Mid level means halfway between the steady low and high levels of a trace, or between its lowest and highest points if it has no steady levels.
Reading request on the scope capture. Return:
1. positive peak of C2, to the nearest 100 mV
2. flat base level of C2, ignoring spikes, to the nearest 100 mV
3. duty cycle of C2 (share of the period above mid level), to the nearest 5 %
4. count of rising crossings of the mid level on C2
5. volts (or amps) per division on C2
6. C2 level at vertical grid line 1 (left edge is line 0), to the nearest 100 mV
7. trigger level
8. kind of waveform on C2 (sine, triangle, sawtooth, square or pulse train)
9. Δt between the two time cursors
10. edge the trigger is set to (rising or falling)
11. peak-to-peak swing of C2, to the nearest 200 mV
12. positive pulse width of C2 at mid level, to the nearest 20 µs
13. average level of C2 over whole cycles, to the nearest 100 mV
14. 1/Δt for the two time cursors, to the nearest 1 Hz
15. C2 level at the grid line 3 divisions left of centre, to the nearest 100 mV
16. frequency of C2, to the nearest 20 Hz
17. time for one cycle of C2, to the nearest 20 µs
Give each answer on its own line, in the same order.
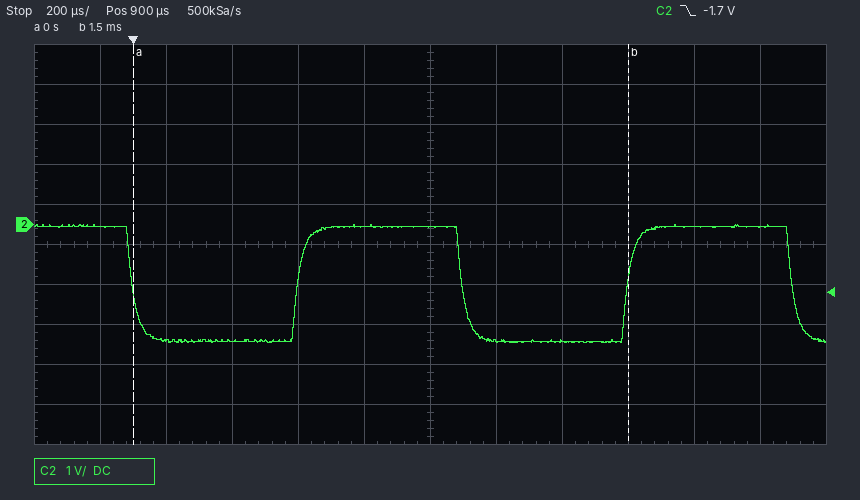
0.0 V
-2.9 V
50 %
2
1 V
0.0 V
-1.7 V
square
1.50 ms
falling
3.0 V
500 µs
-1.5 V
667 Hz
-2.9 V
1.00 kHz
1.00 ms
